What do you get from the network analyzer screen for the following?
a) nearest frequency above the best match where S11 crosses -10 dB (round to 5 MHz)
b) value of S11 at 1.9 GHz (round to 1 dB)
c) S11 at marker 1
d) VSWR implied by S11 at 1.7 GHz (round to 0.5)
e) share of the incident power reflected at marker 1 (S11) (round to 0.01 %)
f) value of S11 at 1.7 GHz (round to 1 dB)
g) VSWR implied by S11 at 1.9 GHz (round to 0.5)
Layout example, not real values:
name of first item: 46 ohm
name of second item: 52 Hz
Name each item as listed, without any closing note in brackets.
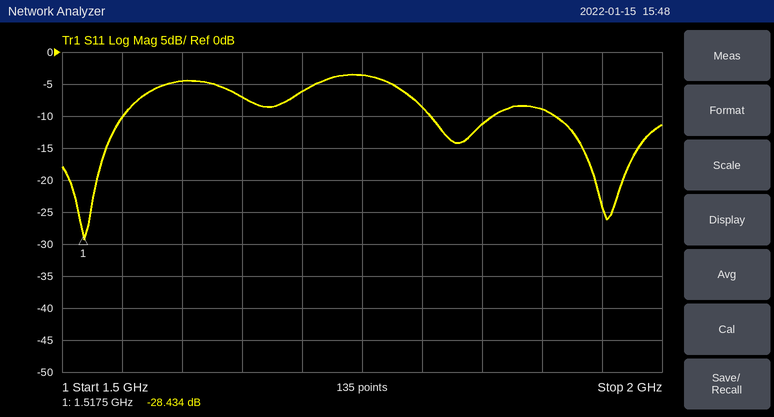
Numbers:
nearest frequency above the best match where S11 crosses -10 dB: 1.550 GHz
value of S11 at 1.9 GHz: -9 dB
S11 at marker 1: -28.434 dB
VSWR implied by S11 at 1.7 GHz: 3.0
share of the incident power reflected at marker 1 (S11): 0.14 %
value of S11 at 1.7 GHz: -6 dB
VSWR implied by S11 at 1.9 GHz: 2.0
